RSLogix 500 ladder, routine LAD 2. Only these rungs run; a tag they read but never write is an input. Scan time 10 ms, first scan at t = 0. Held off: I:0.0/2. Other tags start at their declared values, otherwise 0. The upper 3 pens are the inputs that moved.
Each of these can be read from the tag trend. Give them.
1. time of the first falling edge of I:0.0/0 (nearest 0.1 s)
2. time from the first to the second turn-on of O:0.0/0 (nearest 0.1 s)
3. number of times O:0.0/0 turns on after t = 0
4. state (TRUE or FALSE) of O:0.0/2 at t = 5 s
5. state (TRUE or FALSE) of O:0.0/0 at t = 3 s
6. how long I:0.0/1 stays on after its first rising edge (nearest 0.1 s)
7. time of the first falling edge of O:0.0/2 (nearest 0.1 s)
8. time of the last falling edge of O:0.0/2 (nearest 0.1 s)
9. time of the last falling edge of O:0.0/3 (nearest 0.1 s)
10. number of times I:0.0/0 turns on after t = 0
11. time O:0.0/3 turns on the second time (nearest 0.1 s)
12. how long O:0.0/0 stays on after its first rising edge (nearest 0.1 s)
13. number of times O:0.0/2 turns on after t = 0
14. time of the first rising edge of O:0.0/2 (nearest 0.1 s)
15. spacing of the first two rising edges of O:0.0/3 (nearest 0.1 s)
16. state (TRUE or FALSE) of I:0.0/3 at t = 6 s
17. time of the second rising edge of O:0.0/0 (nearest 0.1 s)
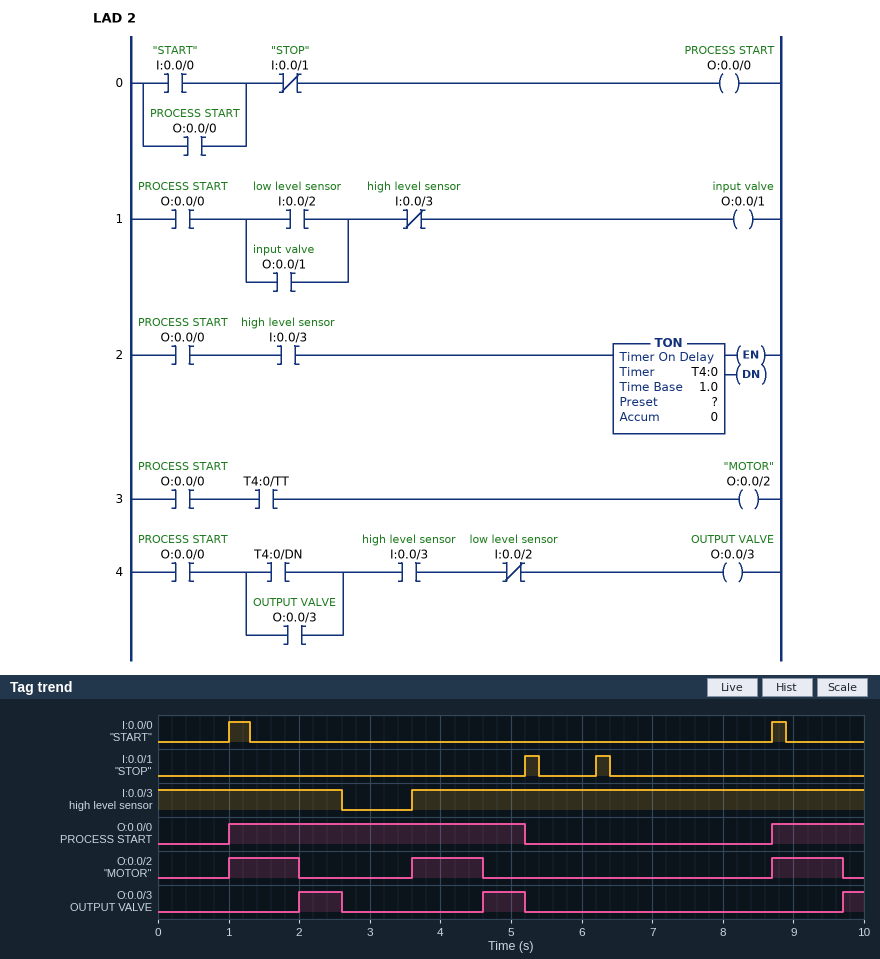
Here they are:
1.3 s
7.7 s
2
FALSE
TRUE
0.2 s
2.0 s
9.7 s
5.2 s
2
4.6 s
4.2 s
3
1.0 s
2.6 s
TRUE
8.7 s
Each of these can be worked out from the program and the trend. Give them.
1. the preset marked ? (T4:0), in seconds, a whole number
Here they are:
1 s
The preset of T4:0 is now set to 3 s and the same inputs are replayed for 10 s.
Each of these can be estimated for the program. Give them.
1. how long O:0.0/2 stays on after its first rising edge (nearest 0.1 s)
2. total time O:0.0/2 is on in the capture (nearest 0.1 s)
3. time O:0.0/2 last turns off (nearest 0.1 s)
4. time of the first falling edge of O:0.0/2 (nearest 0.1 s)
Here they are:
1.6 s
4.5 s
5.2 s
2.6 s
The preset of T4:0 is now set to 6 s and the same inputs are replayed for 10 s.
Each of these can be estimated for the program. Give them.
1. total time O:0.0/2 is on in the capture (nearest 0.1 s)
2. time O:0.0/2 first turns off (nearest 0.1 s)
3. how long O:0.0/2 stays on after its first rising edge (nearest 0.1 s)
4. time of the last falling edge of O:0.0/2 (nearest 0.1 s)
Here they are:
4.5 s
2.6 s
1.6 s
5.2 s
